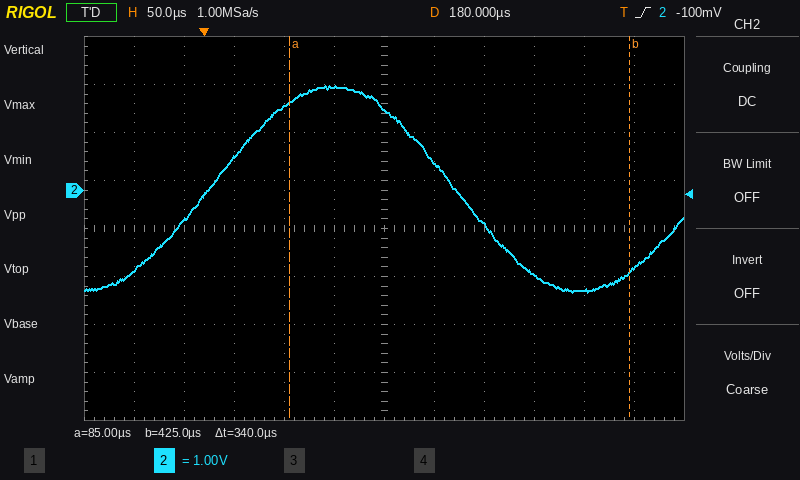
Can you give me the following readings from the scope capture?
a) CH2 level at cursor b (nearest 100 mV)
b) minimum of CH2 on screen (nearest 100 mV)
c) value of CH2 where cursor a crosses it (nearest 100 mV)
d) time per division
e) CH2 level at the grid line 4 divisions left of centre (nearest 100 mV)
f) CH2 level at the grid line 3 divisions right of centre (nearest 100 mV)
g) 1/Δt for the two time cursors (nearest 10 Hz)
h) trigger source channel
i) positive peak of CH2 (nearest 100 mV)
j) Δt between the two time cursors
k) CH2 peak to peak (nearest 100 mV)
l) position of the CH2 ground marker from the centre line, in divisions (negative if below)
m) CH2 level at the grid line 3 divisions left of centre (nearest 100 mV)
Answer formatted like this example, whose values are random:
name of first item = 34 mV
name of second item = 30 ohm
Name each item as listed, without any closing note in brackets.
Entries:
CH2 level at cursor b = -1.7 V
minimum of CH2 on screen = -2.1 V
value of CH2 where cursor a crosses it = 1.8 V
time per division = 50 µs
CH2 level at the grid line 4 divisions left of centre = -600 mV
CH2 level at the grid line 3 divisions right of centre = -1.8 V
1/Δt for the two time cursors = 2.94 kHz
trigger source channel = CH2
positive peak of CH2 = 2.2 V
Δt between the two time cursors = 340 µs
CH2 peak to peak = 4.3 V
position of the CH2 ground marker from the centre line, in divisions = +0.8 div
CH2 level at the grid line 3 divisions left of centre = 700 mV
